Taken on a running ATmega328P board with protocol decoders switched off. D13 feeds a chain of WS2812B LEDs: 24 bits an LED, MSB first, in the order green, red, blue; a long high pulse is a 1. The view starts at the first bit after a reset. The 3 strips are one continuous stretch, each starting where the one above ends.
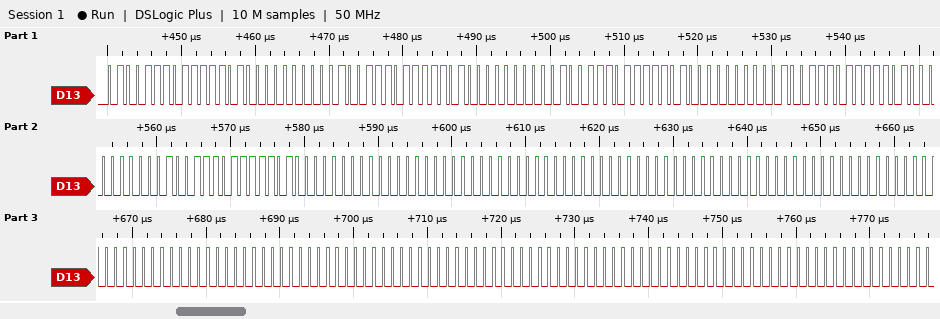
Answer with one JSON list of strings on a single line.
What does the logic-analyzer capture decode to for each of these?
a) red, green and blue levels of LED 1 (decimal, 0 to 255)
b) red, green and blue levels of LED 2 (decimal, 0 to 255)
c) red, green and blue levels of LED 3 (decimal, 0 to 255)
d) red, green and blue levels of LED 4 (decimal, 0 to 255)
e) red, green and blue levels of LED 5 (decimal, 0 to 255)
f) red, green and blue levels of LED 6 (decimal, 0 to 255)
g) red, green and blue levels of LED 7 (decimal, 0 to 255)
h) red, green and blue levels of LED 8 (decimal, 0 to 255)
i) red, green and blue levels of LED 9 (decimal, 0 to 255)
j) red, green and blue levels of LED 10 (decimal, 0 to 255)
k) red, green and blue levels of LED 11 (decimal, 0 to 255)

["250, 78, 0", "250, 78, 0", "250, 78, 0", "250, 78, 0", "250, 78, 0", "0, 0, 0", "0, 0, 0", "0, 0, 0", "0, 0, 0", "0, 0, 0", "0, 0, 0"]
